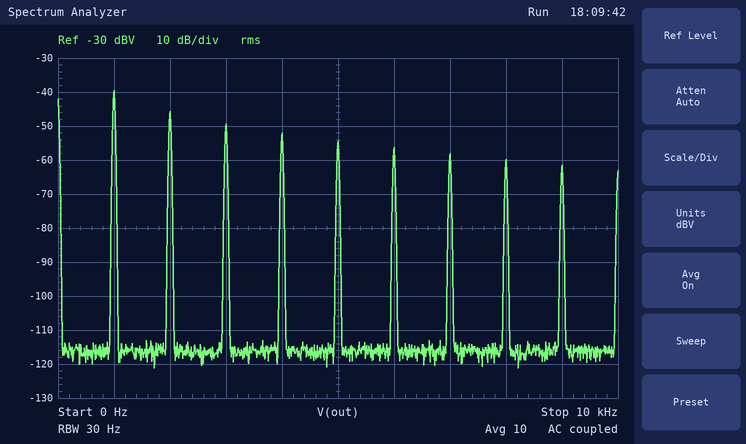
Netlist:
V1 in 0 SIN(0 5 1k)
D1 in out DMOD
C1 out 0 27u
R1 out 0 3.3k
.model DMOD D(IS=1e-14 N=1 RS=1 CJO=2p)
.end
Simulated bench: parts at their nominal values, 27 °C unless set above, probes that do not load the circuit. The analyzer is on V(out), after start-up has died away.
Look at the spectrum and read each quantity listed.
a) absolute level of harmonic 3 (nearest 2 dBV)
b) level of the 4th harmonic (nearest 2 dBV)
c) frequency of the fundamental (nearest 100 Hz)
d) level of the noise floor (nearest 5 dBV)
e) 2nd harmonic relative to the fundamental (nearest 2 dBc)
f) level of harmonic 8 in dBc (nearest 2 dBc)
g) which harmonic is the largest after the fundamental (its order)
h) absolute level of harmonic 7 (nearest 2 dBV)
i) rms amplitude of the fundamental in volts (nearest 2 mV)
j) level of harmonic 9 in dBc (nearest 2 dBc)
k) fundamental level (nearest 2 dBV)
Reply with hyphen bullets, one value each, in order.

- -50 dBV
- -52 dBV
- 1.0 kHz
- -115 dBV
- -6 dBc
- -20 dBc
- 2
- -58 dBV
- 10 mV
- -22 dBc
- -40 dBV
